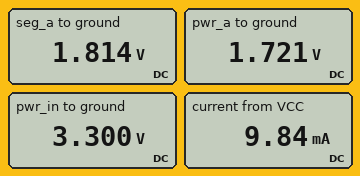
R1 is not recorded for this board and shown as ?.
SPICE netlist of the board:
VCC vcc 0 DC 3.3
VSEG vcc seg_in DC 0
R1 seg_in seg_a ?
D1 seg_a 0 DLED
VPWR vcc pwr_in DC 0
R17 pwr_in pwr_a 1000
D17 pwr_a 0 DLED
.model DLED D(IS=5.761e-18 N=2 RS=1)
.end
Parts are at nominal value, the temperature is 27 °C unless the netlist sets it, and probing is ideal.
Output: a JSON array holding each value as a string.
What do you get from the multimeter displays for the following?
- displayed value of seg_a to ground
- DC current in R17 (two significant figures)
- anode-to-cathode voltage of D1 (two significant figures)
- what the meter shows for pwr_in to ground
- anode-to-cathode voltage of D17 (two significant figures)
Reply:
["1.814 V", "1.6 mA", "1.8 V", "3.300 V", "1.7 V"]
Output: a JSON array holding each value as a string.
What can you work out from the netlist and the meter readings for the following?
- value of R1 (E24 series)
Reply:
["180 Ω"]
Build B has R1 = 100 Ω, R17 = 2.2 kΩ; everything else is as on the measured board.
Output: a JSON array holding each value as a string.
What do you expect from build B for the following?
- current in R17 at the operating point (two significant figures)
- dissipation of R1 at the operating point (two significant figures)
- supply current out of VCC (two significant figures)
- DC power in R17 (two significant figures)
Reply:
["740 µA", "21 mW", "15 mA", "1.2 mW"]
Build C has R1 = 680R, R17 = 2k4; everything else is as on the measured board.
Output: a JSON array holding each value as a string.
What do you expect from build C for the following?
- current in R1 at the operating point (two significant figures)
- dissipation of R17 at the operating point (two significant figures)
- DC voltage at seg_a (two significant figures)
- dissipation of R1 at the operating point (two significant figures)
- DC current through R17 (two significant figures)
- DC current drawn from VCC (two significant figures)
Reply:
["2.3 mA", "1.1 mW", "1.7 V", "3.6 mW", "680 µA", "3.0 mA"]
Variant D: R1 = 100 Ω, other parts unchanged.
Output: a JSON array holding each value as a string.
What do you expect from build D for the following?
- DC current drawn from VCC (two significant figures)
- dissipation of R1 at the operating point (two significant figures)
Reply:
["16 mA", "21 mW"]
